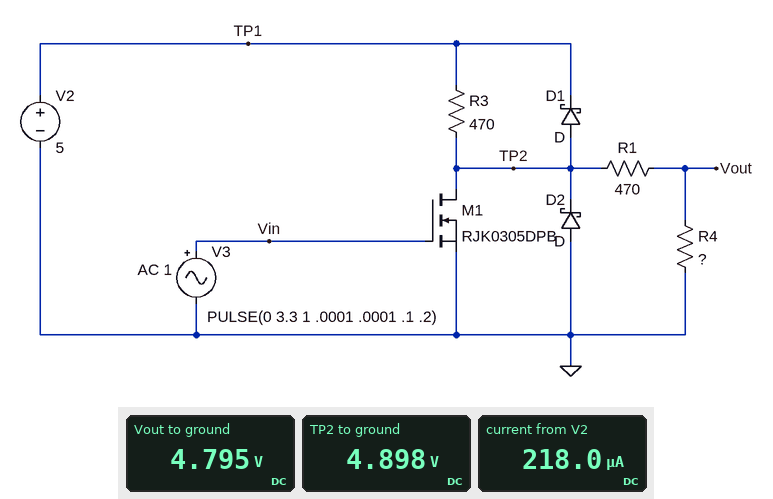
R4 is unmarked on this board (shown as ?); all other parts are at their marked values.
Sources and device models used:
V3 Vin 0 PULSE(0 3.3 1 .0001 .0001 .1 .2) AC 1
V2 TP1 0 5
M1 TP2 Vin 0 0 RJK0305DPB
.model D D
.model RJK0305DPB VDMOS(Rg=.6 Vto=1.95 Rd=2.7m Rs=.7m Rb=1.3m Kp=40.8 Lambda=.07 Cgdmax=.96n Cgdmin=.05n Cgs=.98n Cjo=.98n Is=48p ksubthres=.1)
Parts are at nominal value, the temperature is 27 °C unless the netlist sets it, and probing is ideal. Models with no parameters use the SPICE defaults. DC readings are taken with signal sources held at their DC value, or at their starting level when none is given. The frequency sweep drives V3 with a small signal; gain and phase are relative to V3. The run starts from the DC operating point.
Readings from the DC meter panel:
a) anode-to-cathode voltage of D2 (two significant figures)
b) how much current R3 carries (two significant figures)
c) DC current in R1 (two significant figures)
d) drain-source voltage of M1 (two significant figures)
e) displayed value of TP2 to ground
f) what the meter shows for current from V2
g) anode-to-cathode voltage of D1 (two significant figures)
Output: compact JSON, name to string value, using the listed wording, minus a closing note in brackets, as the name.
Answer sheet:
{"anode-to-cathode voltage of D2": "-4.9 V", "how much current R3 carries": "220 µA", "DC current in R1": "220 µA", "drain-source voltage of M1": "4.9 V", "displayed value of TP2 to ground": "4.898 V", "what the meter shows for current from V2": "218.0 µA", "anode-to-cathode voltage of D1": "-100 mV"}
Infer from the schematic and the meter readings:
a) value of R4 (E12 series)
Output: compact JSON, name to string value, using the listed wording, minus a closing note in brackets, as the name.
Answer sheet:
{"value of R4": "22 kΩ"}
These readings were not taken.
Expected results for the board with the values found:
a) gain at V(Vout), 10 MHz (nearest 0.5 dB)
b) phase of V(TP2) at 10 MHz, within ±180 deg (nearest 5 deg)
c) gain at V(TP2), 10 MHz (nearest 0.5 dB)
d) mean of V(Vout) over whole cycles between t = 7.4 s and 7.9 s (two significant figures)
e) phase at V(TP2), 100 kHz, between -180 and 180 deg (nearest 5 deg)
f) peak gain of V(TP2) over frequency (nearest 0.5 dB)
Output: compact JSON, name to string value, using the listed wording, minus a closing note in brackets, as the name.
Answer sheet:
{"gain at V(Vout), 10 MHz": "-12.5 dB", "phase of V(TP2) at 10 MHz, within ±180 deg": "0 deg", "gain at V(TP2), 10 MHz": "-12.0 dB", "mean of V(Vout) over whole cycles between t = 7.4 s and 7.9 s": "2.4 V", "phase at V(TP2), 100 kHz, between -180 and 180 deg": "80 deg", "peak gain of V(TP2) over frequency": "-12.0 dB"}
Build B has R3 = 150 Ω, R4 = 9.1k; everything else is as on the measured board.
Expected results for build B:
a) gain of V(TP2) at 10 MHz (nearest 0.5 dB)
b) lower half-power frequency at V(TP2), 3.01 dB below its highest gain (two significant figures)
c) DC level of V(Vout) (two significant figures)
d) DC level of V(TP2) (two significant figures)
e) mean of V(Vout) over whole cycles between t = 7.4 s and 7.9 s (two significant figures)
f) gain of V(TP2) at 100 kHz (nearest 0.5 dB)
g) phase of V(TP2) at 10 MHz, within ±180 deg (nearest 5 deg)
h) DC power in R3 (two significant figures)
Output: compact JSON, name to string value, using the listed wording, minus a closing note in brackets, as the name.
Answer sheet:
{"gain of V(TP2) at 10 MHz": "-12.5 dB", "lower half-power frequency at V(TP2), 3.01 dB below its highest gain": "2.2 MHz", "DC level of V(Vout)": "4.7 V", "DC level of V(TP2)": "4.9 V", "mean of V(Vout) over whole cycles between t = 7.4 s and 7.9 s": "2.3 V", "gain of V(TP2) at 100 kHz": "-39.0 dB", "phase of V(TP2) at 10 MHz, within ±180 deg": "10 deg", "DC power in R3": "40 µW"}
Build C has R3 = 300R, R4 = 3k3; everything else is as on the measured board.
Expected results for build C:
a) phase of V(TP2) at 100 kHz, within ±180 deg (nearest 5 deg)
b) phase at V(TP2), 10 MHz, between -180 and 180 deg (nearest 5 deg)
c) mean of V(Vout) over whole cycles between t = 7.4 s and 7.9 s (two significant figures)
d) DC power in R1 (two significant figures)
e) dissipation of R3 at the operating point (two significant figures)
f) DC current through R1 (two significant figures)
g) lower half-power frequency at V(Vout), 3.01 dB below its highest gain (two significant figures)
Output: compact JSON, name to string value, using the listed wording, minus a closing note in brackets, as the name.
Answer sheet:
{"phase of V(TP2) at 100 kHz, within ±180 deg": "85 deg", "phase at V(TP2), 10 MHz, between -180 and 180 deg": "5 deg", "mean of V(Vout) over whole cycles between t = 7.4 s and 7.9 s": "2.0 V", "DC power in R1": "710 µW", "dissipation of R3 at the operating point": "450 µW", "DC current through R1": "1.2 mA", "lower half-power frequency at V(Vout), 3.01 dB below its highest gain": "1.1 MHz"}
